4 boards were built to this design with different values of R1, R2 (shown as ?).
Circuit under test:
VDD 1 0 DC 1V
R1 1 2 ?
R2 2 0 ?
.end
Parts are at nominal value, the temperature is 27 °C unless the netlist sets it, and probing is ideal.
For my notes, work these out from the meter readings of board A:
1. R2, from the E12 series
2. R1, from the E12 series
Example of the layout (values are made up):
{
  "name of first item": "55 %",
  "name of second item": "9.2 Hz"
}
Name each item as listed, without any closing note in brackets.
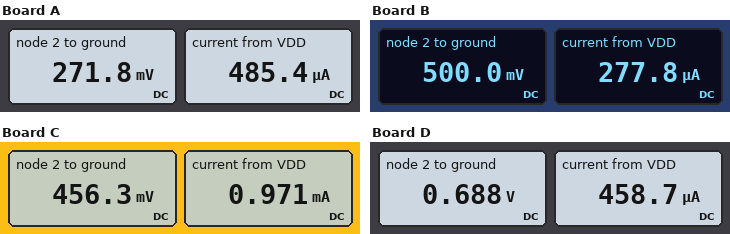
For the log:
{
  "R2, from the E12 series": "560 Ω",
  "R1, from the E12 series": "1.5 kΩ"
}
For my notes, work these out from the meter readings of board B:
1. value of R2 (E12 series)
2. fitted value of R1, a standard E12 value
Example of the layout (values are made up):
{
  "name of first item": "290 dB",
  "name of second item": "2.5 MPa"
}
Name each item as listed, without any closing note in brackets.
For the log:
{
  "value of R2": "1.8 kΩ",
  "fitted value of R1, a standard E12 value": "1.8 kΩ"
}
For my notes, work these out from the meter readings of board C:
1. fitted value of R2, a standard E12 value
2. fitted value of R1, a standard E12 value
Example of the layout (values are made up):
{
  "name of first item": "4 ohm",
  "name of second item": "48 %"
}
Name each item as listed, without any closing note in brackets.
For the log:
{
  "fitted value of R2, a standard E12 value": "470 Ω",
  "fitted value of R1, a standard E12 value": "560 Ω"
}
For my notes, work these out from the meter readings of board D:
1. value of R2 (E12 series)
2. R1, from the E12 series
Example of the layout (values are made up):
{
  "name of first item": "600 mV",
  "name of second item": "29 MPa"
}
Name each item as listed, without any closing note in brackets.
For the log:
{
  "value of R2": "1.5 kΩ",
  "R1, from the E12 series": "680 Ω"
}
